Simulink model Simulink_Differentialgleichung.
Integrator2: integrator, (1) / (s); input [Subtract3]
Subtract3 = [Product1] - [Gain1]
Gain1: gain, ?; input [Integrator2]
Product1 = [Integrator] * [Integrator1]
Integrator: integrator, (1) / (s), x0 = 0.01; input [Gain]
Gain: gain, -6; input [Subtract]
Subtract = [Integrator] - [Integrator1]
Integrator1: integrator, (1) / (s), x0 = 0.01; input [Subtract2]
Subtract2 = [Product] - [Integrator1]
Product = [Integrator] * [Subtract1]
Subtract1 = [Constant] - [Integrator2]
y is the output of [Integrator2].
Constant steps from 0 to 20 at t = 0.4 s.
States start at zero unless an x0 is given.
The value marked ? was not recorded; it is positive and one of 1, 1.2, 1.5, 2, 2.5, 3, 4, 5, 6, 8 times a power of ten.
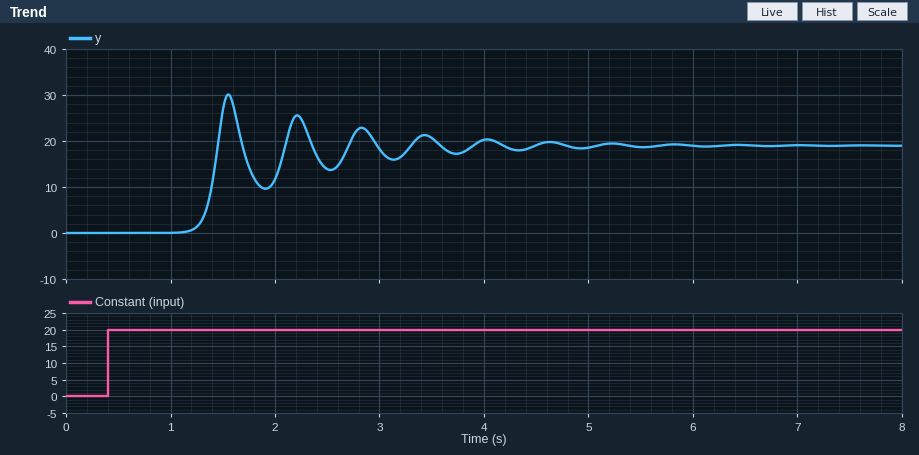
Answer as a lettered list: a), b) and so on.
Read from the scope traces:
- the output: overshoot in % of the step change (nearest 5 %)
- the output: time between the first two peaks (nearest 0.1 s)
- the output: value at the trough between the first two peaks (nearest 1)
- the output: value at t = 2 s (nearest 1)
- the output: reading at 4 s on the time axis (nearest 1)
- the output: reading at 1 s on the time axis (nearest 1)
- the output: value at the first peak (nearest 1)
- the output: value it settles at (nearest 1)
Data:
a) 60 %
b) 0.7 s
c) 10
d) 12
e) 20
f) 0
g) 30
h) 19
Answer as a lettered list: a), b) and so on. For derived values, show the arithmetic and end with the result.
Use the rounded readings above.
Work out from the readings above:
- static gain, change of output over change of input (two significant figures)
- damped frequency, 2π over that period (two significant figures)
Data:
a) (19 - 0) / (20 - 0) = 0.95
b) 2π / 0.7 = 9.0 rad/s
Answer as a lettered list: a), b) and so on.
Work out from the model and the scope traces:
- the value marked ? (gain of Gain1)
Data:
a) 5
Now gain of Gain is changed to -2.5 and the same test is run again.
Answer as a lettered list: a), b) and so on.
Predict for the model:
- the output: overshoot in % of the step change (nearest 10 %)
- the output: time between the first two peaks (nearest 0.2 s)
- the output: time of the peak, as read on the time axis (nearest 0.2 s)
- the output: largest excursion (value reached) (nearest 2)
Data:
a) 50 %
b) 0.6 s
c) 2.0 s
d) 28
